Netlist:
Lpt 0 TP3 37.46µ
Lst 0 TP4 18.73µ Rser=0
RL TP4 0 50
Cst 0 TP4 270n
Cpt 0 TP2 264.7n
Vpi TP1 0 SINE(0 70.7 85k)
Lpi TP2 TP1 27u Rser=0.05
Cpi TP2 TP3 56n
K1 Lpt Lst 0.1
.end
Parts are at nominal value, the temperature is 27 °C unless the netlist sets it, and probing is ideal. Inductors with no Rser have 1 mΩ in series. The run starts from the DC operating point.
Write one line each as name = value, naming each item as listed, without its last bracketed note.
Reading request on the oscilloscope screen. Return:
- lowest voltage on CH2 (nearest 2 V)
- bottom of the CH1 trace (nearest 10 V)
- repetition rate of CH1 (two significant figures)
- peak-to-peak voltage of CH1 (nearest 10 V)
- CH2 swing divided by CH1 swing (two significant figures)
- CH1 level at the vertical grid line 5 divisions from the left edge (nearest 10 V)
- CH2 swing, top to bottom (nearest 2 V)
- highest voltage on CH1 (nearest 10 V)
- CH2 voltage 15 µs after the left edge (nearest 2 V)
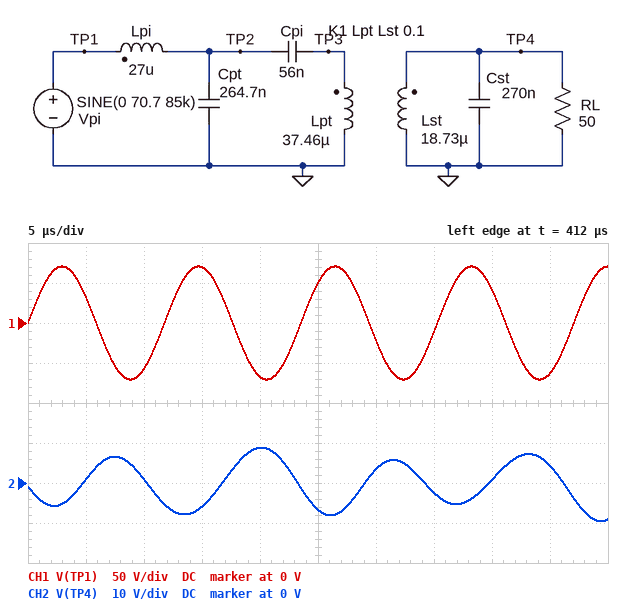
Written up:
lowest voltage on CH2 = -10 V
bottom of the CH1 trace = -70 V
repetition rate of CH1 = 85 kHz
peak-to-peak voltage of CH1 = 140 V
CH2 swing divided by CH1 swing = 0.13
CH1 level at the vertical grid line 5 divisions from the left edge = 50 V
CH2 swing, top to bottom = 18 V
highest voltage on CH1 = 70 V
CH2 voltage 15 µs after the left edge = -6 V
